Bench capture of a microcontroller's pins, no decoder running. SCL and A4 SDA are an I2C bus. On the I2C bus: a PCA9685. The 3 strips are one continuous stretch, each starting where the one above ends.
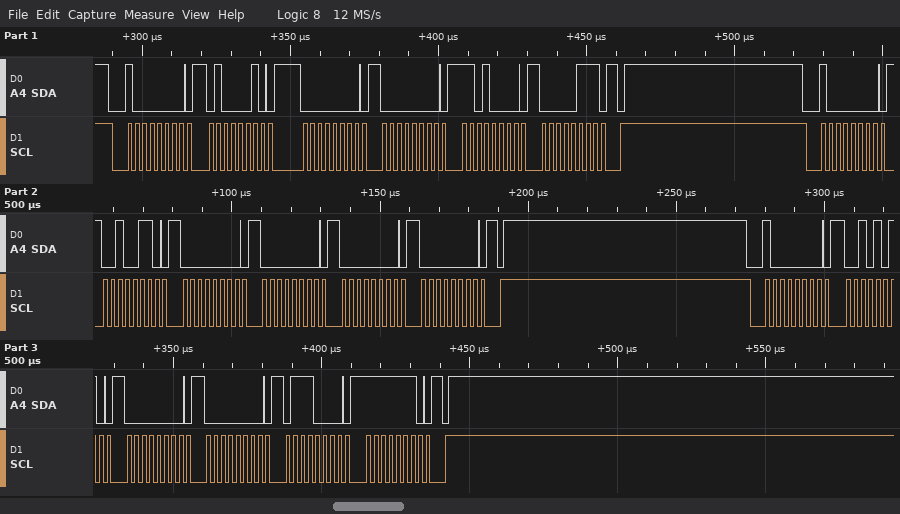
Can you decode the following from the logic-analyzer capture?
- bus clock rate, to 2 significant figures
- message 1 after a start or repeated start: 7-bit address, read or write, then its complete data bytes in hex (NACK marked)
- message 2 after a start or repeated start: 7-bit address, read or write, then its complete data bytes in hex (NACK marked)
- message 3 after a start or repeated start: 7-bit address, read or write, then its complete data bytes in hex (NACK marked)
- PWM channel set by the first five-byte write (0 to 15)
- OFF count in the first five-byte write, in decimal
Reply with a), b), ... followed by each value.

a) 400 kHz
b) 0x40 write: 42 00 00 D0 07
c) 0x40 write: 26 00 00 00 00
d) 0x40 write: 2A 00 00 70 FE
e) 15
f) 2000
